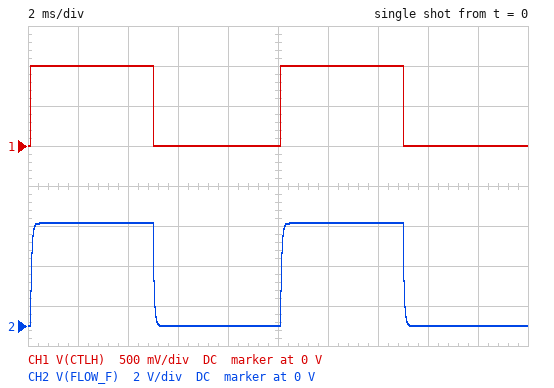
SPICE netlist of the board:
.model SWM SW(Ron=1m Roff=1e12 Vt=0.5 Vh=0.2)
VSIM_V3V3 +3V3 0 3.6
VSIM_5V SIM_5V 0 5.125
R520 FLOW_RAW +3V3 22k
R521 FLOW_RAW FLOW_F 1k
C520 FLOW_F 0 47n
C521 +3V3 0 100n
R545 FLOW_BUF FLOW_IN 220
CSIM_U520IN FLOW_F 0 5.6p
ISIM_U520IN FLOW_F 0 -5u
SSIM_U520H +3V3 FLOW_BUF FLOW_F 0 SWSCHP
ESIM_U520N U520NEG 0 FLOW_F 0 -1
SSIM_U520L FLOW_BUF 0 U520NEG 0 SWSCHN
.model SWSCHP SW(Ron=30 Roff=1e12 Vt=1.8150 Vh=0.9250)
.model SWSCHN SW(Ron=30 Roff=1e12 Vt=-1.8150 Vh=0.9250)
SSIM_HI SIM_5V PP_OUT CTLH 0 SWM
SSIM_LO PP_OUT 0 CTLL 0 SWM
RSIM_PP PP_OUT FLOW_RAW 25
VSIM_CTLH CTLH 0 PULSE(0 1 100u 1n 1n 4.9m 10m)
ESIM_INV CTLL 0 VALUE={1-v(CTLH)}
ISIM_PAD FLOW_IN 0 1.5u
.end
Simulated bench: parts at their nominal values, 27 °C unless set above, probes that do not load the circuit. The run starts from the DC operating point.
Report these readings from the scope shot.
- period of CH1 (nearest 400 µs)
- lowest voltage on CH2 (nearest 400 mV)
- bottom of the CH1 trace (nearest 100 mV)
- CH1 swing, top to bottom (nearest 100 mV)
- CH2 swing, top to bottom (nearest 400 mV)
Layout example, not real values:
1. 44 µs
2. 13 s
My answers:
1. 10.0 ms
2. 0 V
3. 0 V
4. 1.0 V
5. 5.2 V
